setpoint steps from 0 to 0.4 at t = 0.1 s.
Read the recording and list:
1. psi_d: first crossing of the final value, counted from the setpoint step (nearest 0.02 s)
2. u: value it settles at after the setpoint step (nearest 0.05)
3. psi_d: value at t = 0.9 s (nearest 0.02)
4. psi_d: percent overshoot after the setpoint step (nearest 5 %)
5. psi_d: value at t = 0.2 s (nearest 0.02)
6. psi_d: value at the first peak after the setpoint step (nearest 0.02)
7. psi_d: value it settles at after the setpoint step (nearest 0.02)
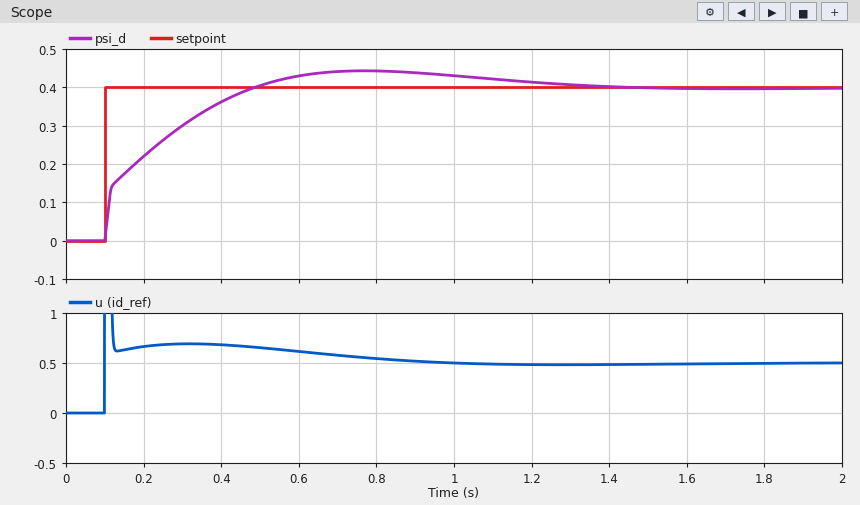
0.38 s
0.50
0.44
10 %
0.22
0.44
0.40
